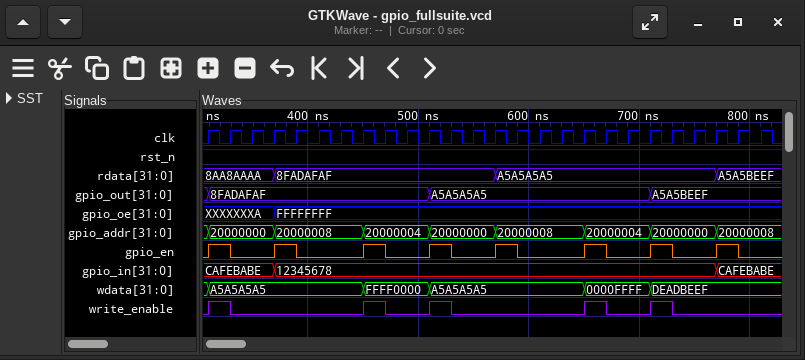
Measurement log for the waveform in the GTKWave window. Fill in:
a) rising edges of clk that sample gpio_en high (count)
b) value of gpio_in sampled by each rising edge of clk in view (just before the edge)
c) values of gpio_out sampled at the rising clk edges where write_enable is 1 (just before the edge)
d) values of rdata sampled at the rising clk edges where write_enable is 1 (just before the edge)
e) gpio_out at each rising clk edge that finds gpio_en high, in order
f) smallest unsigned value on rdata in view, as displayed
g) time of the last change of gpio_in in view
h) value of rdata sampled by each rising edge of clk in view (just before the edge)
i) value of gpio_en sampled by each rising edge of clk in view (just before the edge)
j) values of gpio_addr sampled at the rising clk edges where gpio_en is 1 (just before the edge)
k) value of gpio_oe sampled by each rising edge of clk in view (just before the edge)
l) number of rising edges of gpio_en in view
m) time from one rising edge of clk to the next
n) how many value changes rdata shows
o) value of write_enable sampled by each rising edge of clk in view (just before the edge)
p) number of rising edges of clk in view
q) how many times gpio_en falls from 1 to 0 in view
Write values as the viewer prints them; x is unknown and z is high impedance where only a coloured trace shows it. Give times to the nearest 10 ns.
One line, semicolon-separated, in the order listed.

8; CAFEBABE, CAFEBABE, CAFEBABE, CAFEBABE, 12345678, 12345678, 12345678, 12345678, 12345678, 12345678, 12345678, 12345678, 12345678, 12345678, 12345678, 12345678, 12345678, 12345678, 12345678, 12345678, 12345678, 12345678, 12345678, 12345678, CAFEBABE, CAFEBABE; 8FADAFAF, 8FADAFAF, A5A5A5A5, A5A5A5A5, A5A5BEEF; 8AA8AAAA, 8FADAFAF, 8FADAFAF, A5A5A5A5, A5A5A5A5; 8FADAFAF, 8FADAFAF, 8FADAFAF, A5A5A5A5, A5A5A5A5, A5A5A5A5, A5A5BEEF, A5A5BEEF; 8AA8AAAA; 770 ns; 8AA8AAAA, 8AA8AAAA, 8AA8AAAA, 8AA8AAAA, 8FADAFAF, 8FADAFAF, 8FADAFAF, 8FADAFAF, 8FADAFAF, 8FADAFAF, 8FADAFAF, 8FADAFAF, 8FADAFAF, 8FADAFAF, A5A5A5A5, A5A5A5A5, A5A5A5A5, A5A5A5A5, A5A5A5A5, A5A5A5A5, A5A5A5A5, A5A5A5A5, A5A5A5A5, A5A5A5A5, A5A5BEEF, A5A5BEEF; 0 1 0 0 1 0 0 0 1 0 0 1 0 0 1 0 0 0 1 0 0 1 0 0 1 0; 20000000, 20000008, 20000004, 20000000, 20000008, 20000004, 20000000, 20000008; XXXXXXXA, XXXXXXXA, XXXXXXXA, XXXXXXXA, FFFFFFFF, FFFFFFFF, FFFFFFFF, FFFFFFFF, FFFFFFFF, FFFFFFFF, FFFFFFFF, FFFFFFFF, FFFFFFFF, FFFFFFFF, FFFFFFFF, FFFFFFFF, FFFFFFFF, FFFFFFFF, FFFFFFFF, FFFFFFFF, FFFFFFFF, FFFFFFFF, FFFFFFFF, FFFFFFFF, FFFFFFFF, FFFFFFFF; 8; 20 ns; 3; 0 1 0 0 0 0 0 0 1 0 0 1 0 0 0 0 0 0 1 0 0 1 0 0 0 0; 26; 8
